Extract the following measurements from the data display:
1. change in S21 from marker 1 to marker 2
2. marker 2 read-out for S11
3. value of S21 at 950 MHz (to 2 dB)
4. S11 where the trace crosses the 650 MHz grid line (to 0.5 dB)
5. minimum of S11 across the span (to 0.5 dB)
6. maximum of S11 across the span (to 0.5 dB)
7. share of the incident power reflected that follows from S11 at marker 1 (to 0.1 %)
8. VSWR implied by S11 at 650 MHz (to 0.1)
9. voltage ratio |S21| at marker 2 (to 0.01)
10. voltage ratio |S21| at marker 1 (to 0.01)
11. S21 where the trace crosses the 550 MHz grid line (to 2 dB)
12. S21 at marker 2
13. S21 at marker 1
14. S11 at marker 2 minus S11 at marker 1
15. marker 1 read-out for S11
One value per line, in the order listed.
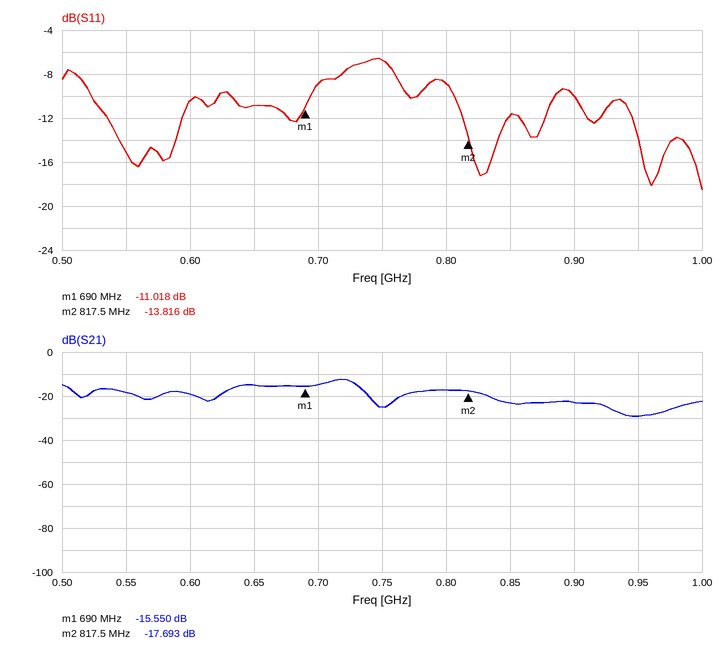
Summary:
-2.143 dB
-13.816 dB
-30 dB
-11.0 dB
-18.5 dB
-6.5 dB
7.9 %
1.8
0.13
0.17
-18 dB
-17.693 dB
-15.550 dB
-2.798 dB
-11.018 dB
